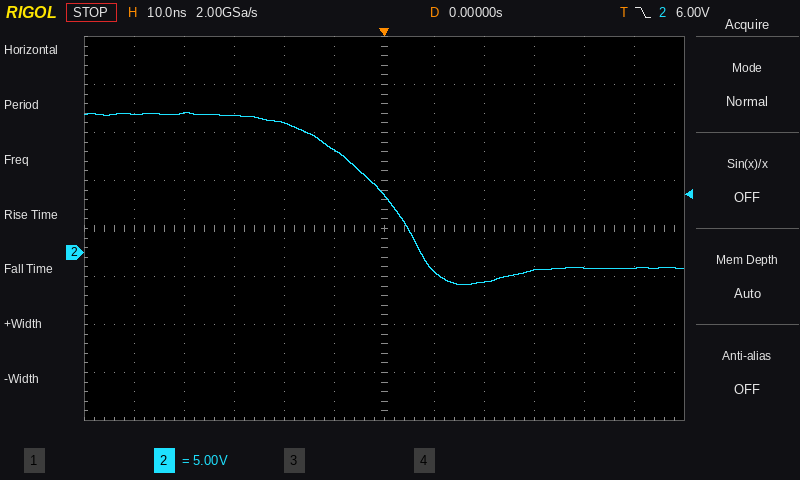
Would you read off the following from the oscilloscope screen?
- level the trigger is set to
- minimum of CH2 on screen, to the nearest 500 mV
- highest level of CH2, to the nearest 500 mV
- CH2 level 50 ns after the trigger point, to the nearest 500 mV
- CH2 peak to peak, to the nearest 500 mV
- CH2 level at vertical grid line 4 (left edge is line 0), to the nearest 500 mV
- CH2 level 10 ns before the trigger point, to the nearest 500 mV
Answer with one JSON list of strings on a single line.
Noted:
["6.00 V", "-3.5 V", "14.5 V", "-1.5 V", "18.0 V", "13.5 V", "10.5 V"]
